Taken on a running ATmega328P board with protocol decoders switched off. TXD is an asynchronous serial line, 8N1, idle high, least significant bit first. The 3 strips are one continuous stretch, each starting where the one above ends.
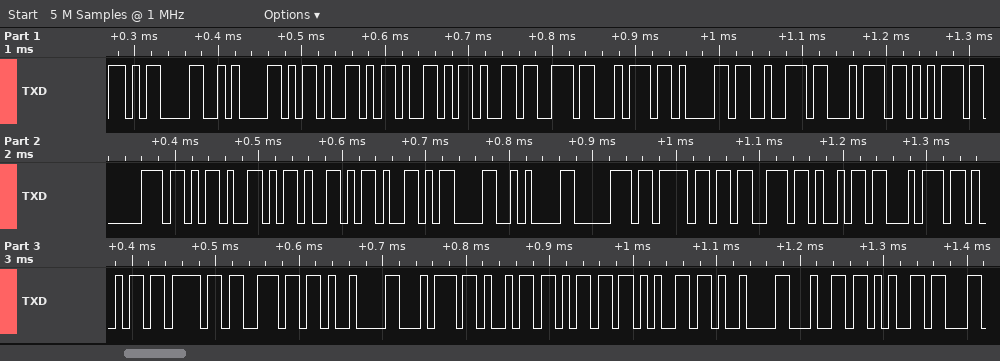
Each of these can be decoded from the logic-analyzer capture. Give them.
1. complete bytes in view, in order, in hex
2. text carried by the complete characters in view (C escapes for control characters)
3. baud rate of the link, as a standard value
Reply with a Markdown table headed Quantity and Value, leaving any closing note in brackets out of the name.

| Quantity | Value |
|---|---|
| complete bytes in view, in order, in hex | 0D 0A 2D 2D 2D 73 74 61 72 74 75 70 2D 2D 2D 0D 0A 70 6F 73 69 74 69 6F 6E 09 74 69 6D 65 09 64 65 |
| text carried by the complete characters in view | "\r\n---startup---\r\nposition\ttime\tde" |
| baud rate of the link, as a standard value | 115200 baud |
